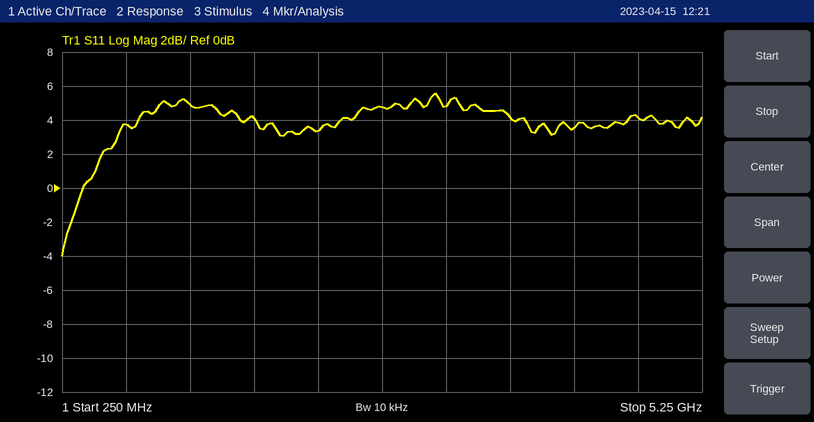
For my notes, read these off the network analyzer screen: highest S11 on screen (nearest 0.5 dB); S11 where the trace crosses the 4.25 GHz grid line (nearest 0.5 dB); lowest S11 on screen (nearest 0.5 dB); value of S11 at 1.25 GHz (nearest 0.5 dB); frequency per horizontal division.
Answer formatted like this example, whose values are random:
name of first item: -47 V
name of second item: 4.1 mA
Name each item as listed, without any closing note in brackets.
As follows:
highest S11 on screen: 5.5 dB
S11 where the trace crosses the 4.25 GHz grid line: 3.5 dB
lowest S11 on screen: -4.0 dB
value of S11 at 1.25 GHz: 5.0 dB
frequency per horizontal division: 500 MHz
